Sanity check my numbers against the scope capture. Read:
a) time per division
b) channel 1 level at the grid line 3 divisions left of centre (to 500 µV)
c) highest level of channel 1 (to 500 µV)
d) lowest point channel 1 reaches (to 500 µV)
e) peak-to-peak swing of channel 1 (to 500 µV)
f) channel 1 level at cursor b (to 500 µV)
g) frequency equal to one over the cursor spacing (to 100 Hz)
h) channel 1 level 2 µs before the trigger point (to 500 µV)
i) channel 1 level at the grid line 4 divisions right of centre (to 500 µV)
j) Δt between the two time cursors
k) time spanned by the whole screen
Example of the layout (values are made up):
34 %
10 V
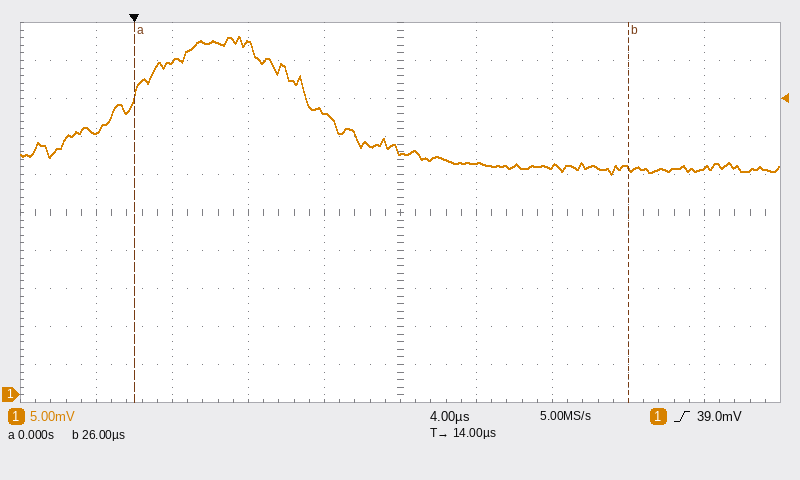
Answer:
4 µs
44.0 mV
47.0 mV
29.0 mV
18.0 mV
30.0 mV
38.5 kHz
34.5 mV
30.0 mV
26.0 µs
40 µs
